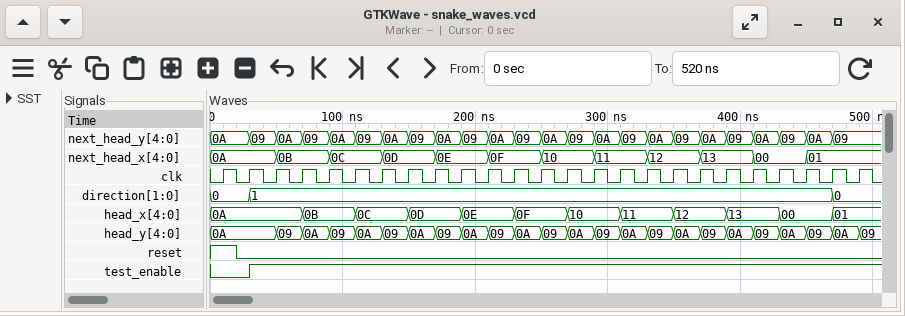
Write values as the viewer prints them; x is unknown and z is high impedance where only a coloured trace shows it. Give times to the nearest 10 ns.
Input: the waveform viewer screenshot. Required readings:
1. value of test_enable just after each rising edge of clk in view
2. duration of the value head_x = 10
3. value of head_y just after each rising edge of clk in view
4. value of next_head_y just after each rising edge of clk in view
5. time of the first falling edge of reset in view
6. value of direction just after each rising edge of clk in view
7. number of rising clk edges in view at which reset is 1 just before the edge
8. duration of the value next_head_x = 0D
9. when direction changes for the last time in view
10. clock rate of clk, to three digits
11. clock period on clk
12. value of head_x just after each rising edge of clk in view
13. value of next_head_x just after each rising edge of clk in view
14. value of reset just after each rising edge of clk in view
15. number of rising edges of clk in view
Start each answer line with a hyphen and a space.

- 0 1 1 1 1 1 1 1 1 1 1 1 1 1 1 1 1 1 1 1 1 1 1 1 1
- 40 ns
- 0A, 0A, 09, 0A, 09, 0A, 09, 0A, 09, 0A, 09, 0A, 09, 0A, 09, 0A, 09, 0A, 09, 0A, 09, 0A, 09, 0A, 09
- 0A, 09, 0A, 09, 0A, 09, 0A, 09, 0A, 09, 0A, 09, 0A, 09, 0A, 09, 0A, 09, 0A, 09, 0A, 09, 0A, 09, 09
- 20 ns
- 0, 1, 1, 1, 1, 1, 1, 1, 1, 1, 1, 1, 1, 1, 1, 1, 1, 1, 1, 1, 1, 1, 1, 0, 0
- 1
- 40 ns
- 470 ns
- 50.0 MHz
- 20 ns
- 0A, 0A, 0A, 0B, 0B, 0C, 0C, 0D, 0D, 0E, 0E, 0F, 0F, 10, 10, 11, 11, 12, 12, 13, 13, 00, 00, 01, 01
- 0A, 0A, 0B, 0B, 0C, 0C, 0D, 0D, 0E, 0E, 0F, 0F, 10, 10, 11, 11, 12, 12, 13, 13, 00, 00, 01, 01, 01
- 1 0 0 0 0 0 0 0 0 0 0 0 0 0 0 0 0 0 0 0 0 0 0 0 0
- 25
